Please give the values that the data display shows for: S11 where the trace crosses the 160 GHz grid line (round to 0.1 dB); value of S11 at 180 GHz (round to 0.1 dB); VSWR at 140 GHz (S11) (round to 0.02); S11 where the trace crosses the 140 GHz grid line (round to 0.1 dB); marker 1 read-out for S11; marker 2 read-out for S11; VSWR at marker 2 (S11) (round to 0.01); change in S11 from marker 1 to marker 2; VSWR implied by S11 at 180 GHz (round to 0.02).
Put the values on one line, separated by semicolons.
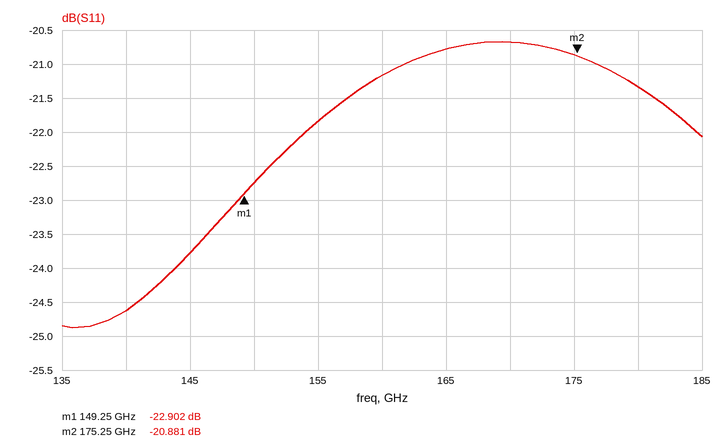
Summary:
-21.2 dB; -21.3 dB; 1.12; -24.6 dB; -22.902 dB; -20.881 dB; 1.20; 2.021 dB; 1.18
